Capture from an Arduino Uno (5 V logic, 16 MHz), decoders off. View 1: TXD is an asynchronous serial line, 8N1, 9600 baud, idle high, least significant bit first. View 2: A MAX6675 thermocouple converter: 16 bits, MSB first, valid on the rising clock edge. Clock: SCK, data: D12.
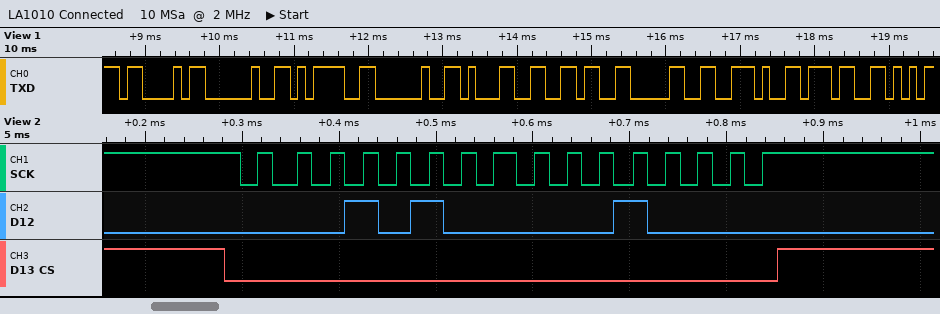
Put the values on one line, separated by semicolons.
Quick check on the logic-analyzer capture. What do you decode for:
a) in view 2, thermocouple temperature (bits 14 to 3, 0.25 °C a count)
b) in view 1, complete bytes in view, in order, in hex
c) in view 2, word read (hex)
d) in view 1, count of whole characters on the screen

160.50 °C; 43 20 3D 20 31 36 30 2E 37; 0x1410; 9
